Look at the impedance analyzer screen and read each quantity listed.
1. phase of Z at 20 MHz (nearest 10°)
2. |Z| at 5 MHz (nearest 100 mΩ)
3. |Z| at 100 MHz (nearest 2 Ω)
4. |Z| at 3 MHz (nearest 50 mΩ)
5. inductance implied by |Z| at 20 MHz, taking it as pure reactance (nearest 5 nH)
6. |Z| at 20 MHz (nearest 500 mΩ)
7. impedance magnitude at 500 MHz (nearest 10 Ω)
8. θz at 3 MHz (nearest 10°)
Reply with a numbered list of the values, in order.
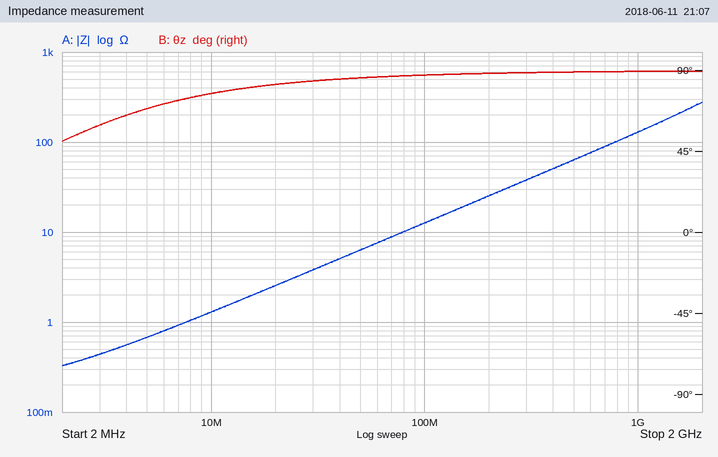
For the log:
1. 80°
2. 700 mΩ
3. 12 Ω
4. 450 mΩ
5. 20 nH
6. 2.5 Ω
7. 60 Ω
8. 60°
